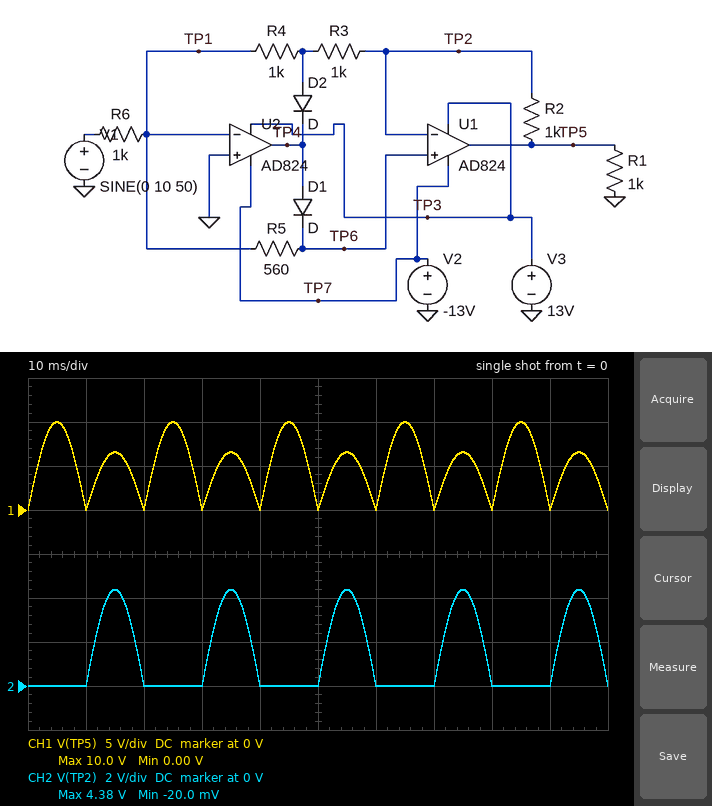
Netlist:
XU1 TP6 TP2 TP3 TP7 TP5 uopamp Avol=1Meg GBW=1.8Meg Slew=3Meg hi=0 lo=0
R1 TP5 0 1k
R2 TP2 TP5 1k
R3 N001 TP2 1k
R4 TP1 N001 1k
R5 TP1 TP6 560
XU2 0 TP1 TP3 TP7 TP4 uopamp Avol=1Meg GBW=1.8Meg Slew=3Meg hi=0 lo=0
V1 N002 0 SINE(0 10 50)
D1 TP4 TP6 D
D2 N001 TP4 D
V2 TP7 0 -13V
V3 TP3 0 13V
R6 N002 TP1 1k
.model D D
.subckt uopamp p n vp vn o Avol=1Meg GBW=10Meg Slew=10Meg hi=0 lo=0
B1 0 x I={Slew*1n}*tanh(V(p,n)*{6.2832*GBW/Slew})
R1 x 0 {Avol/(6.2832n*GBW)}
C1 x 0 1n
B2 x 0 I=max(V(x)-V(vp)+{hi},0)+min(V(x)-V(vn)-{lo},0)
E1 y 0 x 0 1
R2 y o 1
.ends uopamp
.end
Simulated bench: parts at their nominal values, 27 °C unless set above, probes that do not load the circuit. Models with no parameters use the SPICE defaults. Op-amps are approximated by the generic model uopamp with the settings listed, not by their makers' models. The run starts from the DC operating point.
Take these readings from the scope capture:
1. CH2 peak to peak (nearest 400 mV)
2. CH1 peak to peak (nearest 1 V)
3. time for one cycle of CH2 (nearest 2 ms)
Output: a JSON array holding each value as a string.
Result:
["4.4 V", "10 V", "20 ms"]
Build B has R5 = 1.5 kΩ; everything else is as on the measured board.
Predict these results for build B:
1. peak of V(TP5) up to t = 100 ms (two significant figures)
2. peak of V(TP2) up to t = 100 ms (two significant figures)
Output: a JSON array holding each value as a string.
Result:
["13 V", "8.6 V"]
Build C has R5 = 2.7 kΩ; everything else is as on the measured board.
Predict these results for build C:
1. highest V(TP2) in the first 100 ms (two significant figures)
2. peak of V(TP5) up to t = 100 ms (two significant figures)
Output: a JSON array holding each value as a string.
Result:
["8.7 V", "13 V"]
